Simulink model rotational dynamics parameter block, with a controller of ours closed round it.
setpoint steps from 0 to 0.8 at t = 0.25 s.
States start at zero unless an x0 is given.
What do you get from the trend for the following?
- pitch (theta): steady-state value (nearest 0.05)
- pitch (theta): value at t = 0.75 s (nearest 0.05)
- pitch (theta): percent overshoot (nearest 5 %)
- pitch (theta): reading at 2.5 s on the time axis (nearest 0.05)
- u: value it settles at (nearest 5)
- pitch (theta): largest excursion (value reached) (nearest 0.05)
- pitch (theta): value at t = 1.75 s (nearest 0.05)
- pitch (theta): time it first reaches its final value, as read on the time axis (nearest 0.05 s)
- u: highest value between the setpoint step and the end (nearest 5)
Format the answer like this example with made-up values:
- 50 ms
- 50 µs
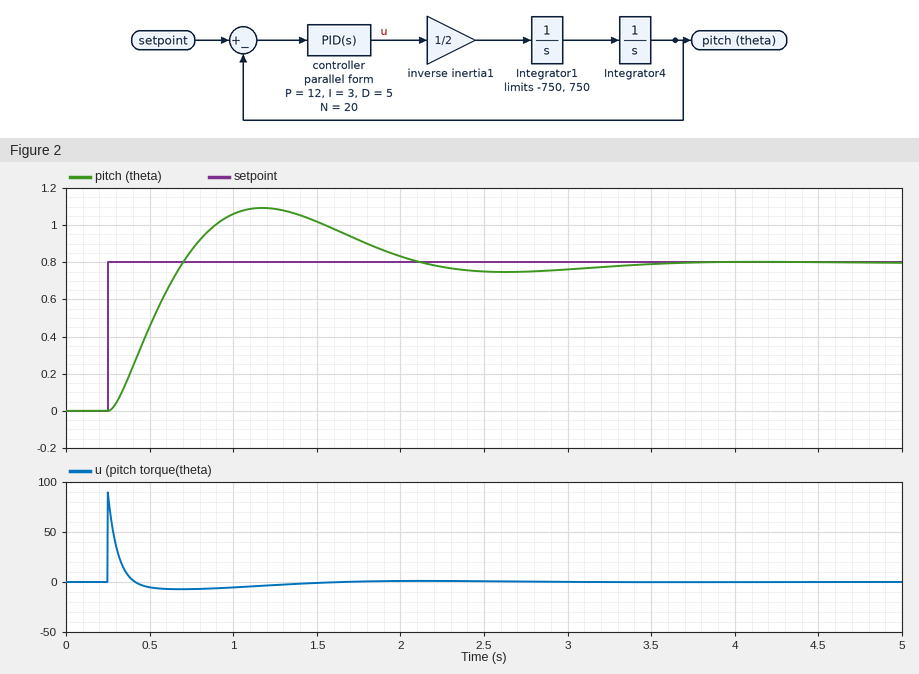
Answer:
- 0.80
- 0.85
- 35 %
- 0.75
- 0
- 1.10
- 0.90
- 0.70 s
- 90
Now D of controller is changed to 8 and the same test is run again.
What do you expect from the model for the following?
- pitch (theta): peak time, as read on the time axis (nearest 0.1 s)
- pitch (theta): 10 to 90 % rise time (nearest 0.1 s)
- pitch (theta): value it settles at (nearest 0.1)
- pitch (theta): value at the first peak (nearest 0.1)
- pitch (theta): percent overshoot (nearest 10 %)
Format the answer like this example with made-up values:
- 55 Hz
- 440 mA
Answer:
- 1.0 s
- 0.3 s
- 0.8
- 1.0
- 20 %
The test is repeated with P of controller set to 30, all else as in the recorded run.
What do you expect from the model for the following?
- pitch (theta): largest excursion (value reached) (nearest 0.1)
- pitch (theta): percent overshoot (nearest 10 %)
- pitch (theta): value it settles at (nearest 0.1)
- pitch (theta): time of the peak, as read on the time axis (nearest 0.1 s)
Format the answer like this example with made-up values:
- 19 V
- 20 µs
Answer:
- 1.2
- 50 %
- 0.8
- 0.9 s
